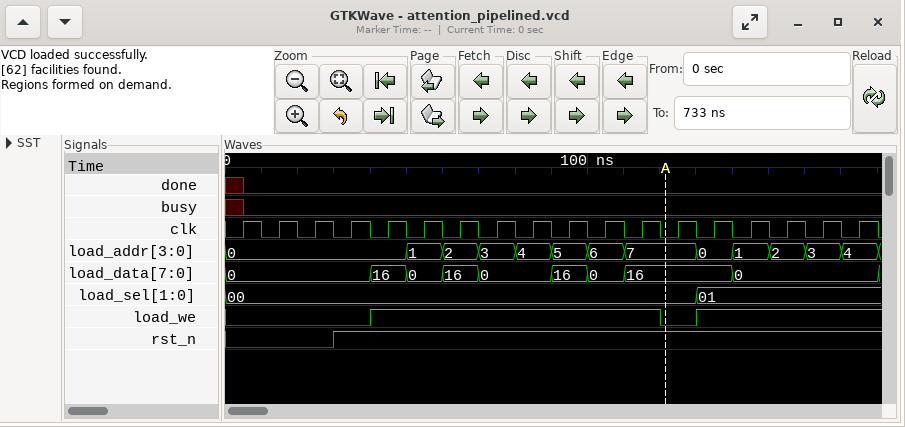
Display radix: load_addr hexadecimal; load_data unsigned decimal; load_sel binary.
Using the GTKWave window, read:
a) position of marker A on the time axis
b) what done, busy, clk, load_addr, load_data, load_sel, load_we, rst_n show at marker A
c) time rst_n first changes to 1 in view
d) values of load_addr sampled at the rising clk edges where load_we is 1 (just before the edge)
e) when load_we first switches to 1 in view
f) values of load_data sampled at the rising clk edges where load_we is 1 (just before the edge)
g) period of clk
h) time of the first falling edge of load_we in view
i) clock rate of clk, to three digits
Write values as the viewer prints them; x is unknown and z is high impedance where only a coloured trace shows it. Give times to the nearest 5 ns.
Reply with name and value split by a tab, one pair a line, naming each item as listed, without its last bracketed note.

position of marker A on the time axis	120 ns
what done, busy, clk, load_addr, load_data, load_sel, load_we, rst_n show at marker A	done=0, busy=0, clk=0, load_addr=7, load_data=16, load_sel=00, load_we=0, rst_n=1
time rst_n first changes to 1 in view	30 ns
values of load_addr sampled at the rising clk edges where load_we is 1	0, 1, 2, 3, 4, 5, 6, 7, 0, 1, 2, 3, 4
when load_we first switches to 1 in view	40 ns
values of load_data sampled at the rising clk edges where load_we is 1	16, 0, 16, 0, 0, 16, 0, 16, 16, 0, 0, 0, 0
period of clk	10 ns
time of the first falling edge of load_we in view	120 ns
clock rate of clk, to three digits	100 MHz
